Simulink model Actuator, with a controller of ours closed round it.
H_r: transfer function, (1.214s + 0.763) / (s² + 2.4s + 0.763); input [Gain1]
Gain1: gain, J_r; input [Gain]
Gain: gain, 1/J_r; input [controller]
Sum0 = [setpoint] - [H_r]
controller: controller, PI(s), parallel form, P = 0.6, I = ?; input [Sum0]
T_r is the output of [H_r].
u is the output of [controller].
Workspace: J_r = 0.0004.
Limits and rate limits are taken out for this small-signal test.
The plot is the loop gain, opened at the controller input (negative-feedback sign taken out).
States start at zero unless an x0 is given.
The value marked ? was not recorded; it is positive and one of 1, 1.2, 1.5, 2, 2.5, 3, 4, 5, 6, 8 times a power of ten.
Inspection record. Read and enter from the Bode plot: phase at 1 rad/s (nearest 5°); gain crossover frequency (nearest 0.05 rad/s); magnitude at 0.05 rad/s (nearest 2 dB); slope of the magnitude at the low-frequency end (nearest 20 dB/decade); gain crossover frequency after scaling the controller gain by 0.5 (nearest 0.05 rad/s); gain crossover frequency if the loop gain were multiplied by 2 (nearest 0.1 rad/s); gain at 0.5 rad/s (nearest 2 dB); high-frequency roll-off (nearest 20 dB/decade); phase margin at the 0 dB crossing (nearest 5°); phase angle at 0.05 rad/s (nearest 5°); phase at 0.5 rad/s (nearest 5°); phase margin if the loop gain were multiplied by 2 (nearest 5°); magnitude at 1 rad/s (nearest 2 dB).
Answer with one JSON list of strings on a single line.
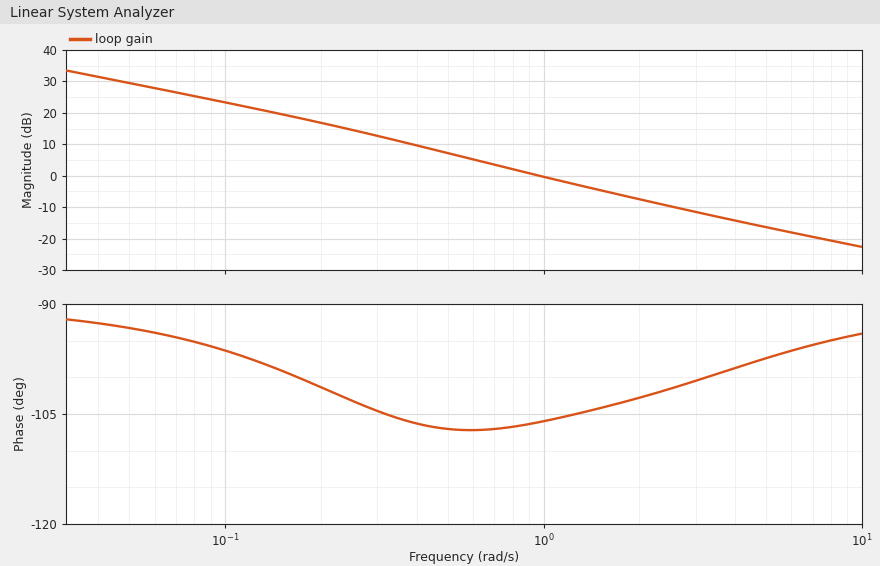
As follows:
["-105°", "0.95 rad/s", "30 dB", "-20 dB/decade", "0.55 rad/s", "1.7 rad/s", "8 dB", "-20 dB/decade", "75°", "-95°", "-105°", "75°", "0 dB"]
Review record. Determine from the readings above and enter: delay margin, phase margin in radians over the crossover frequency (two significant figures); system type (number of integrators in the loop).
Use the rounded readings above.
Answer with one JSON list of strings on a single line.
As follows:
["1.4 s", "1"]
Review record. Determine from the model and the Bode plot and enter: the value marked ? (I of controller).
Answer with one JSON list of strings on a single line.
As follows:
["1.5"]
